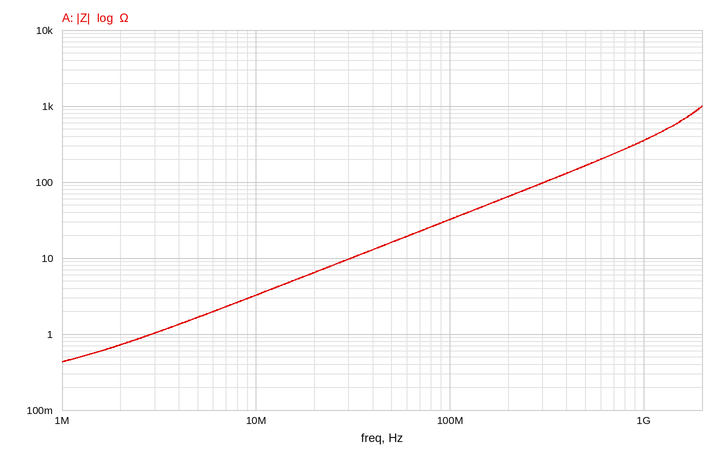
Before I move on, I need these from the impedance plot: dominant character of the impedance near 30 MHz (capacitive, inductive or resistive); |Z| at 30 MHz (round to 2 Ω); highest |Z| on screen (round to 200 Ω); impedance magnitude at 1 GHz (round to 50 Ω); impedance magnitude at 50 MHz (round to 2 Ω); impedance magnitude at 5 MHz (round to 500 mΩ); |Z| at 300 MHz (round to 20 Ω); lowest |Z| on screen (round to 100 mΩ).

inductive
10 Ω
1.0 kΩ
350 Ω
16 Ω
1.5 Ω
100 Ω
400 mΩ
